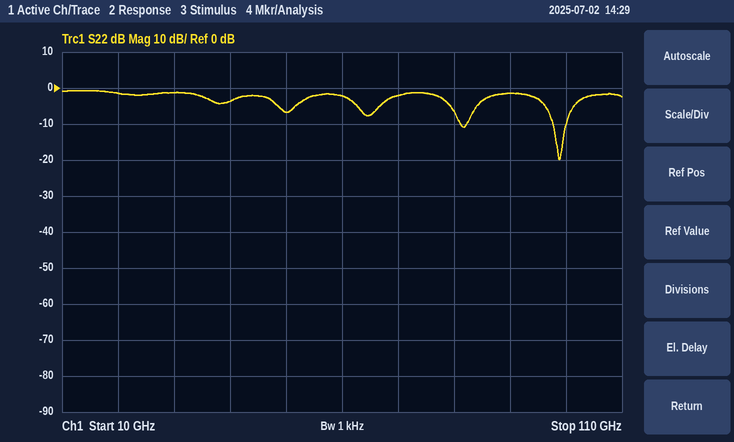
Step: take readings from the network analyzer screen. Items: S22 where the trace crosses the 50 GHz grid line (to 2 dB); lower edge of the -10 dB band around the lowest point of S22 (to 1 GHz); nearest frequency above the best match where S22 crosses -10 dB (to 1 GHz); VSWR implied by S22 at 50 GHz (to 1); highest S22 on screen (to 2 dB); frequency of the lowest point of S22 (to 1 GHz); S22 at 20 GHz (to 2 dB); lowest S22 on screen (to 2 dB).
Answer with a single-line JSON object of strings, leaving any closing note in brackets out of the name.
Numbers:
{"S22 where the trace crosses the 50 GHz grid line": "-6 dB", "lower edge of the -10 dB band around the lowest point of S22": "98 GHz", "nearest frequency above the best match where S22 crosses -10 dB": "100 GHz", "VSWR implied by S22 at 50 GHz": "3", "highest S22 on screen": "0 dB", "frequency of the lowest point of S22": "99 GHz", "S22 at 20 GHz": "-2 dB", "lowest S22 on screen": "-20 dB"}
